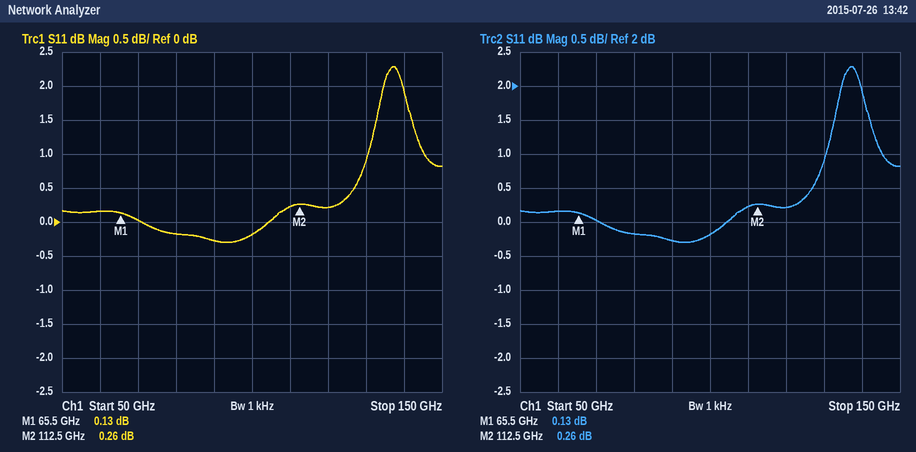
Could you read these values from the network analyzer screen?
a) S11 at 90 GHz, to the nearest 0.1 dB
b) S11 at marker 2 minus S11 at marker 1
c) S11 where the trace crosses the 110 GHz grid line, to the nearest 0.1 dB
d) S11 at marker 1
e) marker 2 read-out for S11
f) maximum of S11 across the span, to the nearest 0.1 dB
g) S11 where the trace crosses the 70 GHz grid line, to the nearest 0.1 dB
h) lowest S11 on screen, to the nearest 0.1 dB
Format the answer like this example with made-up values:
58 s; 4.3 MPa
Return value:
-0.3 dB; 0.13 dB; 0.2 dB; 0.13 dB; 0.26 dB; 2.3 dB; 0.0 dB; -0.3 dB
